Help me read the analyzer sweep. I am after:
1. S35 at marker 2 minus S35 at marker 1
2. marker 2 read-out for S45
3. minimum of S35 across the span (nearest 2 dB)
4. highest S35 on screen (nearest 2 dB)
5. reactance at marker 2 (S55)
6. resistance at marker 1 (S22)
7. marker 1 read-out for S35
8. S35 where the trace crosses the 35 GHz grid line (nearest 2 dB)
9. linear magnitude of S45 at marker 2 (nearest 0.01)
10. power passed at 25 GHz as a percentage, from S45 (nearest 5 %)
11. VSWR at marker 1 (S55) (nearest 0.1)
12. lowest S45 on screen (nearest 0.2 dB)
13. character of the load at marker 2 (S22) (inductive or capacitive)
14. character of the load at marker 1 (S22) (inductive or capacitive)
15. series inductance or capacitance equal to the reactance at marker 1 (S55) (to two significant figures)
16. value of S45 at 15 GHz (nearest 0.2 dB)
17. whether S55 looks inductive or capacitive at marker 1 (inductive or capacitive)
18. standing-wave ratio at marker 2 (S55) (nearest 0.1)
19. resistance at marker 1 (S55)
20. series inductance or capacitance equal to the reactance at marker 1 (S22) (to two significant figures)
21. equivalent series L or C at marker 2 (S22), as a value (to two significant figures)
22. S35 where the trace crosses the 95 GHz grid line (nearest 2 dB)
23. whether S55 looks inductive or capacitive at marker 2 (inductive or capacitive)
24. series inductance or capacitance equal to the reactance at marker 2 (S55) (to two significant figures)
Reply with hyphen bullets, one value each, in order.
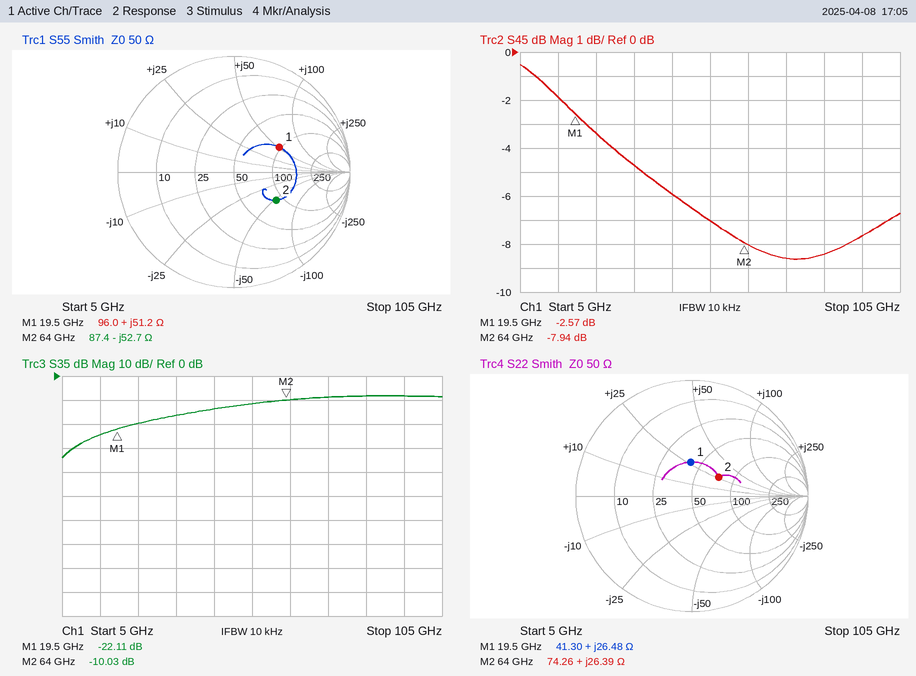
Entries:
- 12.08 dB
- -7.94 dB
- -34 dB
- -8 dB
- -52.7 Ω
- 41.30 Ω
- -22.11 dB
- -16 dB
- 0.40
- 45 %
- 2.6
- -8.6 dB
- inductive
- inductive
- 420 pH
- -1.8 dB
- inductive
- 2.6
- 96.0 Ω
- 220 pH
- 66 pH
- -8 dB
- capacitive
- 47 fF
